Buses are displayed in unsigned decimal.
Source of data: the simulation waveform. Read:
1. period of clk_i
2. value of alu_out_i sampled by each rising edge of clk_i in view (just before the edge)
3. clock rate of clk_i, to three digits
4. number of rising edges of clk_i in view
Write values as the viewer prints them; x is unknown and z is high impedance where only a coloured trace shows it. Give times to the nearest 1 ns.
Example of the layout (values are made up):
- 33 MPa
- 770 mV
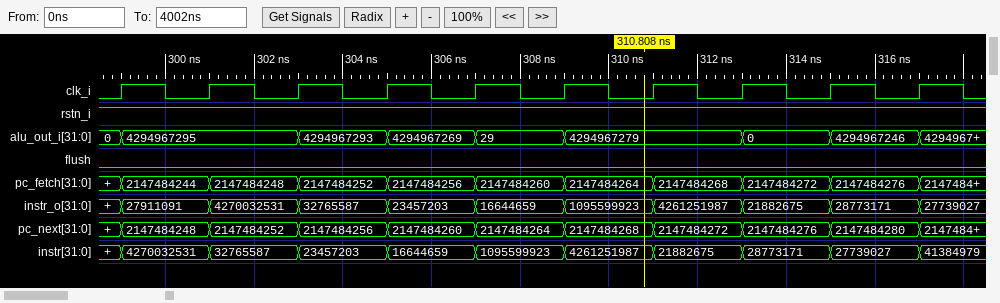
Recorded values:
- 2 ns
- 0, 4294967295, 4294967295, 4294967293, 4294967269, 29, 4294967279, 4294967279, 0, 4294967246
- 500 MHz
- 10
